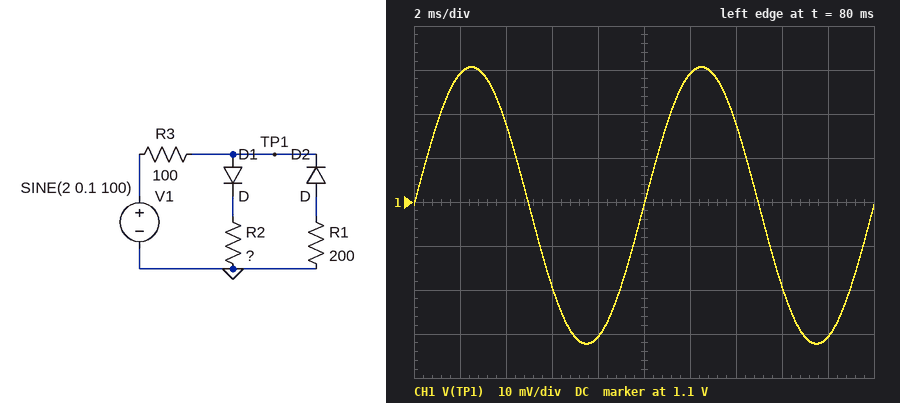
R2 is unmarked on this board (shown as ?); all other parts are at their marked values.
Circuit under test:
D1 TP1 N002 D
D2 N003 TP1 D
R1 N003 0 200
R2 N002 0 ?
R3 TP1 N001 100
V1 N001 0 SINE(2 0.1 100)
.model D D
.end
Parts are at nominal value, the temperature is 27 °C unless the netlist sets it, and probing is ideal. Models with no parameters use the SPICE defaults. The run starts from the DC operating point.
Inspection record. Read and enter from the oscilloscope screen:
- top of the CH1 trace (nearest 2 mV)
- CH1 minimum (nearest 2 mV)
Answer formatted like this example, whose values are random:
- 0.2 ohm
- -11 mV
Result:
- 1.130 V
- 1.068 V
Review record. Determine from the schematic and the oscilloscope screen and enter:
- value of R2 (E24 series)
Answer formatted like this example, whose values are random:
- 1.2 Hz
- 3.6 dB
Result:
- 43 Ω
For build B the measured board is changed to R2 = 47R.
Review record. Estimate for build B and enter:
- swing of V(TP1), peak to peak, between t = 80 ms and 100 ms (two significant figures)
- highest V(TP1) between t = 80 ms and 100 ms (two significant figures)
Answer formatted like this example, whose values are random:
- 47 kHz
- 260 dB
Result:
- 67 mV
- 1.2 V
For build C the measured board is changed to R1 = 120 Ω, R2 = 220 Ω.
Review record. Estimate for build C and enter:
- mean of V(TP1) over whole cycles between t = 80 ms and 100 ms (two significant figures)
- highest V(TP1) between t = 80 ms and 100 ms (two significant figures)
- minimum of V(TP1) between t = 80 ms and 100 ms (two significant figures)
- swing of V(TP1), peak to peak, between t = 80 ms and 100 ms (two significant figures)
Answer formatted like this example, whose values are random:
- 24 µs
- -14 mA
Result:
- 1.6 V
- 1.7 V
- 1.5 V
- 140 mV
